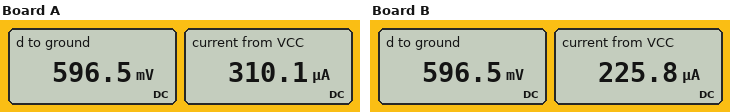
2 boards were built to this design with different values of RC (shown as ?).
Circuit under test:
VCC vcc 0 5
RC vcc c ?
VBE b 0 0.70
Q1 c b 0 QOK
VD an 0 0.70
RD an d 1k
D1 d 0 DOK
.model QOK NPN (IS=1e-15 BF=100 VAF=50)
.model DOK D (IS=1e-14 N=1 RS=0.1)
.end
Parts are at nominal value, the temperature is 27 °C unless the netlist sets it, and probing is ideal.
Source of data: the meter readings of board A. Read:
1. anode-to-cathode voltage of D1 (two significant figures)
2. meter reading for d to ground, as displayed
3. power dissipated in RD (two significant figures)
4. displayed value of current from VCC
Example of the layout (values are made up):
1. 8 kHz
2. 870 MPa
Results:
1. 600 mV
2. 596.5 mV
3. 11 µW
4. 310.1 µA
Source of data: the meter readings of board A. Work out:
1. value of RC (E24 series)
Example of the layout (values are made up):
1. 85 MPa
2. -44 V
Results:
1. 16 kΩ
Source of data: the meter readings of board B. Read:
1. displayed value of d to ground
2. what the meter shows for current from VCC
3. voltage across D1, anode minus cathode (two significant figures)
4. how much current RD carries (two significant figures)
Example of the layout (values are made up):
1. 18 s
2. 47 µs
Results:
1. 596.5 mV
2. 225.8 µA
3. 600 mV
4. 100 µA
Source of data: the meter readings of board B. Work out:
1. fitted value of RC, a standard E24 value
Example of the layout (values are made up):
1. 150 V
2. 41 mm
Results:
1. 22 kΩ
